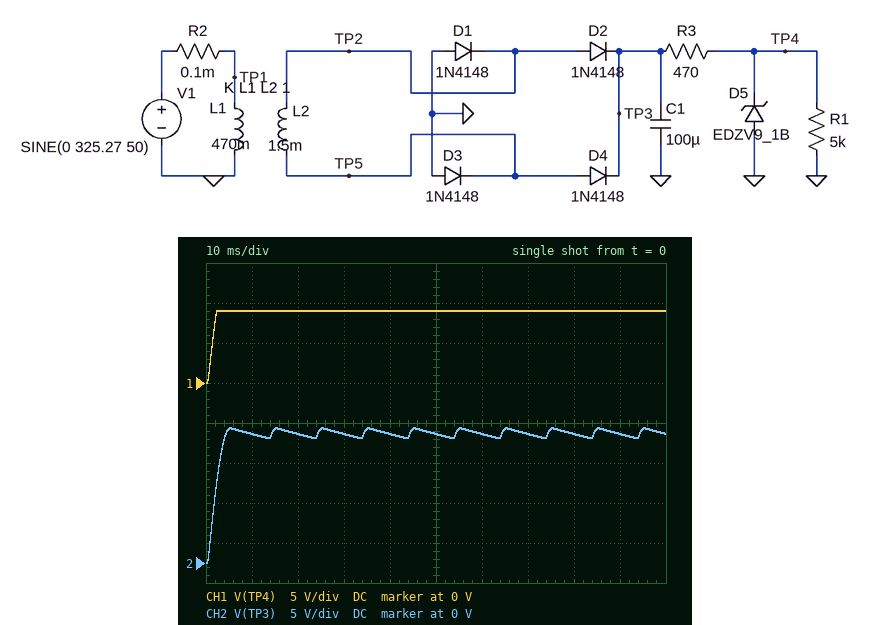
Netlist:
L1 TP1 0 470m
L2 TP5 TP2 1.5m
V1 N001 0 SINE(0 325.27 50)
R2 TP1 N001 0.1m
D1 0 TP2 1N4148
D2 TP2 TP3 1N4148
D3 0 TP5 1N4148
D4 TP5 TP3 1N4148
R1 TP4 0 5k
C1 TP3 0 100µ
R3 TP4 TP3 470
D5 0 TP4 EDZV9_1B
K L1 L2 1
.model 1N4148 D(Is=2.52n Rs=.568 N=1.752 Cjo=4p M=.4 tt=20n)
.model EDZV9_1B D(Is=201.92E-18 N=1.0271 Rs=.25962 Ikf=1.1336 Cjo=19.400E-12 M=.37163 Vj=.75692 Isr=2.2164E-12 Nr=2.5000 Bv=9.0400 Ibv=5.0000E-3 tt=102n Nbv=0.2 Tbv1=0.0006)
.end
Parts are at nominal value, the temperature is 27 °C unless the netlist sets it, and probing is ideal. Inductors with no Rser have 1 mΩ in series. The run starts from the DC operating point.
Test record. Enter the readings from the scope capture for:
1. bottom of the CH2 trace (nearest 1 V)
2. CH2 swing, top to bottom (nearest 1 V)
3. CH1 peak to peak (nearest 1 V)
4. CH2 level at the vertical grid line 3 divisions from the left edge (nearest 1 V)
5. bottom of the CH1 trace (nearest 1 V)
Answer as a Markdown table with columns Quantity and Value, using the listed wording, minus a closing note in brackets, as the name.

| Quantity | Value |
|---|---|
| bottom of the CH2 trace | 0 V |
| CH2 swing, top to bottom | 17 V |
| CH1 peak to peak | 9 V |
| CH2 level at the vertical grid line 3 divisions from the left edge | 16 V |
| bottom of the CH1 trace | 0 V |
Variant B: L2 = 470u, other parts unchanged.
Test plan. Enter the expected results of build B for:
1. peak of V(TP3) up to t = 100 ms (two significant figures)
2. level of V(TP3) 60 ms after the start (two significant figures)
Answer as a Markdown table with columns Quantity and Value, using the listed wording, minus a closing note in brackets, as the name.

| Quantity | Value |
|---|---|
| peak of V(TP3) up to t = 100 ms | 8.9 V |
| level of V(TP3) 60 ms after the start | 8.8 V |
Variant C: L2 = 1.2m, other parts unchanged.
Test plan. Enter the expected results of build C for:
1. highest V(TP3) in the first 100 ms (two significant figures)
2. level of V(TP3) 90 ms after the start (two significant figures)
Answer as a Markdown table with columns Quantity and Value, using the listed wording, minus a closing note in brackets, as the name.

| Quantity | Value |
|---|---|
| highest V(TP3) in the first 100 ms | 15 V |
| level of V(TP3) 90 ms after the start | 14 V |
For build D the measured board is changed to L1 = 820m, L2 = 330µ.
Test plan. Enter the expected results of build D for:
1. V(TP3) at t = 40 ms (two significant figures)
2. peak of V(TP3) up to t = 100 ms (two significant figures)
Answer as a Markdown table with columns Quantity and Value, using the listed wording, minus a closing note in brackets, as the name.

| Quantity | Value |
|---|---|
| V(TP3) at t = 40 ms | 5.1 V |
| peak of V(TP3) up to t = 100 ms | 5.2 V |
